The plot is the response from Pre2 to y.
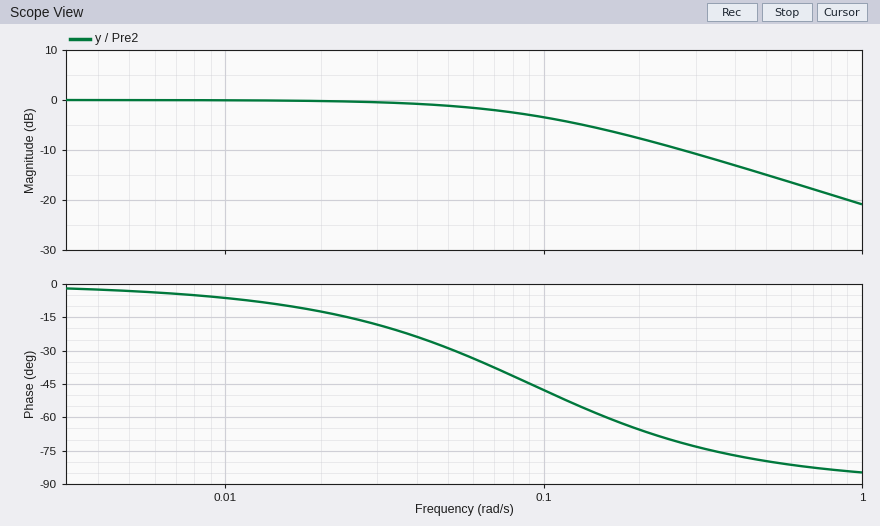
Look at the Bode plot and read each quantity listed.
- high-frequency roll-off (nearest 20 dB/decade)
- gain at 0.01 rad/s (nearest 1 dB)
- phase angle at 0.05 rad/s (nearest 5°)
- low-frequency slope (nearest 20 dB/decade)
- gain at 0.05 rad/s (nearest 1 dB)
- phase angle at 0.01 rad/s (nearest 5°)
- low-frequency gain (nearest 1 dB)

-20 dB/decade
0 dB
-30°
0 dB/decade
-1 dB
-5°
0 dB
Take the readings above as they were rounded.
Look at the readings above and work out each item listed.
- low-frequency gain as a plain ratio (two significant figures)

1.0
